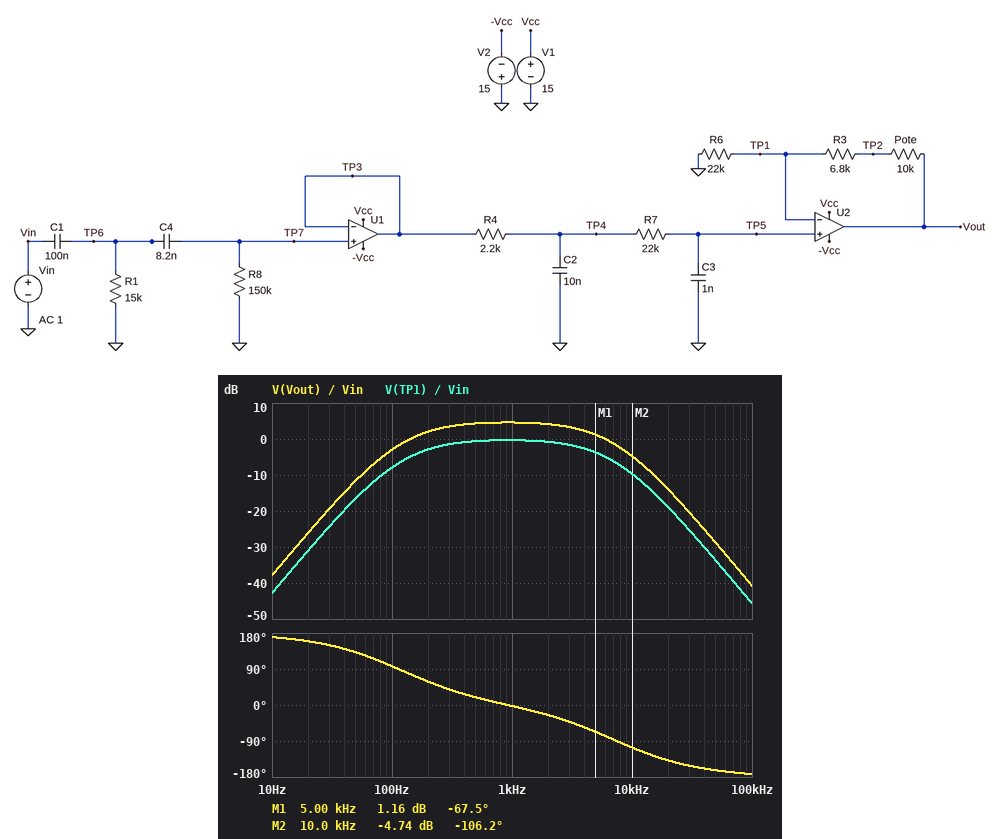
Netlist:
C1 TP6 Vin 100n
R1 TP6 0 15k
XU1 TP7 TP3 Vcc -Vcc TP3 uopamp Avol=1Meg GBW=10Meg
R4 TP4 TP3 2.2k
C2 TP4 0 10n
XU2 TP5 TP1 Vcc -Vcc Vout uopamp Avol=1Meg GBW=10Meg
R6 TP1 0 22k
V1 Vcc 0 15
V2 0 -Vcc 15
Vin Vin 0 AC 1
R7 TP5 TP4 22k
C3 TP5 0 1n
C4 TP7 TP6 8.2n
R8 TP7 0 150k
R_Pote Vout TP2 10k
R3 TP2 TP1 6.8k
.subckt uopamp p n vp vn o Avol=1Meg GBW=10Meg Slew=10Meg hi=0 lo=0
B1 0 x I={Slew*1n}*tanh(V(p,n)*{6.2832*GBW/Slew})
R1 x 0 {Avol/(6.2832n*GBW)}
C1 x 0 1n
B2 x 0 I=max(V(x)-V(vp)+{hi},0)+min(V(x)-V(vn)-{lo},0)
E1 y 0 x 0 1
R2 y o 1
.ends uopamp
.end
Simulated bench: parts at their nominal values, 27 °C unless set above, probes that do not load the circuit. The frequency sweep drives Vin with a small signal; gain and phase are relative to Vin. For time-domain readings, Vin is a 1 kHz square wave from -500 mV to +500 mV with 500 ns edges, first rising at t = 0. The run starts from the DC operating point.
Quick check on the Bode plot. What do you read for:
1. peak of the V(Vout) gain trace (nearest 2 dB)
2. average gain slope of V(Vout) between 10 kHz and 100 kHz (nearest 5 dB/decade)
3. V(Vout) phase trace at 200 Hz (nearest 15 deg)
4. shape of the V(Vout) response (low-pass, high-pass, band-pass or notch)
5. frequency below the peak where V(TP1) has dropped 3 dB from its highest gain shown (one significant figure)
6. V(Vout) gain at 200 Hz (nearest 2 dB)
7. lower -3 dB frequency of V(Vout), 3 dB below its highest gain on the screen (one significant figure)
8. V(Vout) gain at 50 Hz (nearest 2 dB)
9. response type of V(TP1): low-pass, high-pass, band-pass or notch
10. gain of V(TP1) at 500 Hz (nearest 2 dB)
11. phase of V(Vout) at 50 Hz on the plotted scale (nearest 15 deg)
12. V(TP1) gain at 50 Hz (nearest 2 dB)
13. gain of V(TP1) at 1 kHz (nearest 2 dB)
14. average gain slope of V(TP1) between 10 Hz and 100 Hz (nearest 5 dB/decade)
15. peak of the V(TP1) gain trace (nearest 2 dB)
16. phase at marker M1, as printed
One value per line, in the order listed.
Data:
4 dB
-35 dB/decade
60 deg
band-pass
200 Hz
2 dB
200 Hz
-12 dB
band-pass
0 dB
135 deg
-16 dB
0 dB
35 dB/decade
0 dB
-67.5 deg
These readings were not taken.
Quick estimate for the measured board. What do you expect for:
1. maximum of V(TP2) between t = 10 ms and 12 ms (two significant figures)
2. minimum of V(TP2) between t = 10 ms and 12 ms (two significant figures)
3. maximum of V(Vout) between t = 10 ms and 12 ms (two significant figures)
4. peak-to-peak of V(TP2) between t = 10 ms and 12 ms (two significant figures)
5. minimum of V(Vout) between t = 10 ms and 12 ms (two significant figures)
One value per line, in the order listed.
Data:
760 mV
-760 mV
1.0 V
1.5 V
-1.0 V
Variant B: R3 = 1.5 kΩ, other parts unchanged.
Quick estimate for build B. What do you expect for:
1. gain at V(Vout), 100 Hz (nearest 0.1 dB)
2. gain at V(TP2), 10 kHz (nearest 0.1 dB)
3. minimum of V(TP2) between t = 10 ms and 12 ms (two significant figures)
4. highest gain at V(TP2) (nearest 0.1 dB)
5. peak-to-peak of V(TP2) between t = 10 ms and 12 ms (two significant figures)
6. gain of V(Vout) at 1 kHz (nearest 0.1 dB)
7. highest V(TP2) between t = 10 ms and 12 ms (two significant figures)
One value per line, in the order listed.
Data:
-4.3 dB
-9.1 dB
-620 mV
0.2 dB
1.2 V
3.3 dB
620 mV
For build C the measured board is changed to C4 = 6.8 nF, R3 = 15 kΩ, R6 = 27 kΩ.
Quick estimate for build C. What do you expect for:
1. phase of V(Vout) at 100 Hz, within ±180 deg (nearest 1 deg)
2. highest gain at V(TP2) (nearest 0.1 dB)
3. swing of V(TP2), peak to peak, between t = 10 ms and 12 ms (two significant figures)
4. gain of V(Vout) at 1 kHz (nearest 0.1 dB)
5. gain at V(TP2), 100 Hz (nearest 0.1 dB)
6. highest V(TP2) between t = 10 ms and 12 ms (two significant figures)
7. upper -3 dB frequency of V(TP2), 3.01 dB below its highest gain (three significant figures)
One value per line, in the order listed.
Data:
102 deg
3.5 dB
1.8 V
5.3 dB
-5.1 dB
910 mV
4.67 kHz
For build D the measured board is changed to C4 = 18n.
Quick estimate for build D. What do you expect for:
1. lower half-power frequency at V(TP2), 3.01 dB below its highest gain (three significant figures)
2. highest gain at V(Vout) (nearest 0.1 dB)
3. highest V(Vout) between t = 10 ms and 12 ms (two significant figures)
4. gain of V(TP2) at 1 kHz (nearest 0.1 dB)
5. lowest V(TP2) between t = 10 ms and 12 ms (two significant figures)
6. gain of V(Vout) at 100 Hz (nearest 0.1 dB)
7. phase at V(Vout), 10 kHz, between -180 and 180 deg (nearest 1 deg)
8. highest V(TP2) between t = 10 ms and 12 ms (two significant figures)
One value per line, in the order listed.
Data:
135 Hz
4.7 dB
960 mV
2.1 dB
-740 mV
-0.2 dB
-107 deg
710 mV
